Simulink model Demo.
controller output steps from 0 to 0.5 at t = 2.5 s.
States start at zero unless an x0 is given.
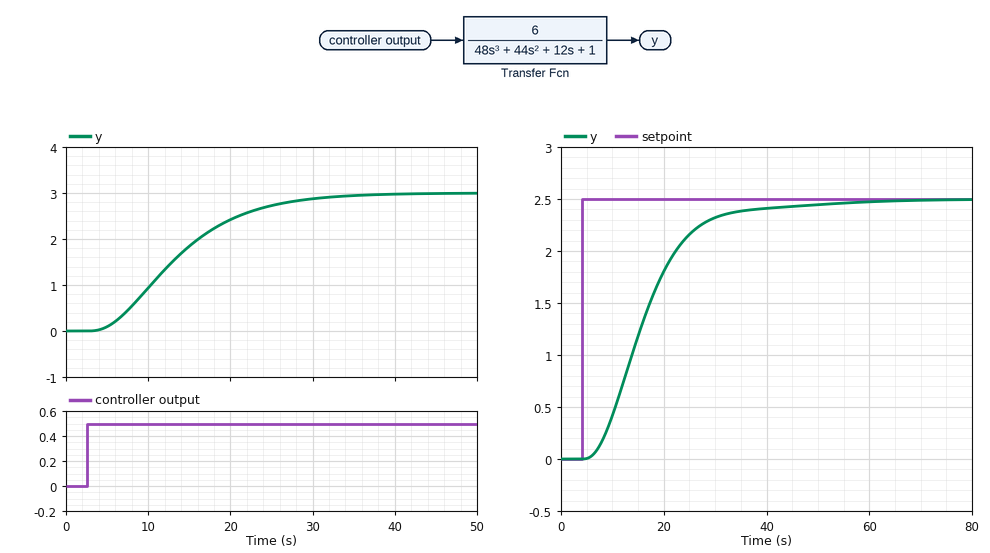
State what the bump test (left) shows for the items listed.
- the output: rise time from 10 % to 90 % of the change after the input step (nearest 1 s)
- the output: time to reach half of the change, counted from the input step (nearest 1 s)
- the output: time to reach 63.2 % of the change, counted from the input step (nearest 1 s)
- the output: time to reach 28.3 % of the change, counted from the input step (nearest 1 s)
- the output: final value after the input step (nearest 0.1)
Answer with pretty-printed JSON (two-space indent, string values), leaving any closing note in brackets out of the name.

{
  "the output: rise time from 10 % to 90 % of the change after the input step": "18 s",
  "the output: time to reach half of the change, counted from the input step": "10 s",
  "the output: time to reach 63.2 % of the change, counted from the input step": "13 s",
  "the output: time to reach 28.3 % of the change, counted from the input step": "7 s",
  "the output: final value after the input step": "3.0"
}
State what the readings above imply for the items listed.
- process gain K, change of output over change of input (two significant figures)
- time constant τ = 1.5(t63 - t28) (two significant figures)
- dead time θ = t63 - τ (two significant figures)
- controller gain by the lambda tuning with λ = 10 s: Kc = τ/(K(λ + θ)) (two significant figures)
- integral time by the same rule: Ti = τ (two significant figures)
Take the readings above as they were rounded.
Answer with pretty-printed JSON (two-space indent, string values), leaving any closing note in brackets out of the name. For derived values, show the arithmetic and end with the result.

{
  "process gain K, change of output over change of input": "(3 - 0) / 0.5 = 6.0",
  "time constant τ = 1.5(t63 - t28)": "1.5 × (13 - 7) = 9.0 s",
  "dead time θ = t63 - τ": "13 - 9 = 4.0 s",
  "controller gain by the lambda tuning with λ = 10 s: Kc = τ/(K(λ + θ))": "9 / (6 × (10 + 4)) = 0.11",
  "integral time by the same rule: Ti = τ": "9.0 s"
}
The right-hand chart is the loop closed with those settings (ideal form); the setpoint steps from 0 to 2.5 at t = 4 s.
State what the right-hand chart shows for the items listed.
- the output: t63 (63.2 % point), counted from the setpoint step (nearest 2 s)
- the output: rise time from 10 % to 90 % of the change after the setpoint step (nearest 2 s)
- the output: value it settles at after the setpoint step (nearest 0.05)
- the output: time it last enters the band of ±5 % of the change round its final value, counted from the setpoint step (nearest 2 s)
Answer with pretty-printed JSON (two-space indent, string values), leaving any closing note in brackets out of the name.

{
  "the output: t63 (63.2 % point), counted from the setpoint step": "14 s",
  "the output: rise time from 10 % to 90 % of the change after the setpoint step": "18 s",
  "the output: value it settles at after the setpoint step": "2.50",
  "the output: time it last enters the band of ±5 % of the change round its final value, counted from the setpoint step": "30 s"
}
